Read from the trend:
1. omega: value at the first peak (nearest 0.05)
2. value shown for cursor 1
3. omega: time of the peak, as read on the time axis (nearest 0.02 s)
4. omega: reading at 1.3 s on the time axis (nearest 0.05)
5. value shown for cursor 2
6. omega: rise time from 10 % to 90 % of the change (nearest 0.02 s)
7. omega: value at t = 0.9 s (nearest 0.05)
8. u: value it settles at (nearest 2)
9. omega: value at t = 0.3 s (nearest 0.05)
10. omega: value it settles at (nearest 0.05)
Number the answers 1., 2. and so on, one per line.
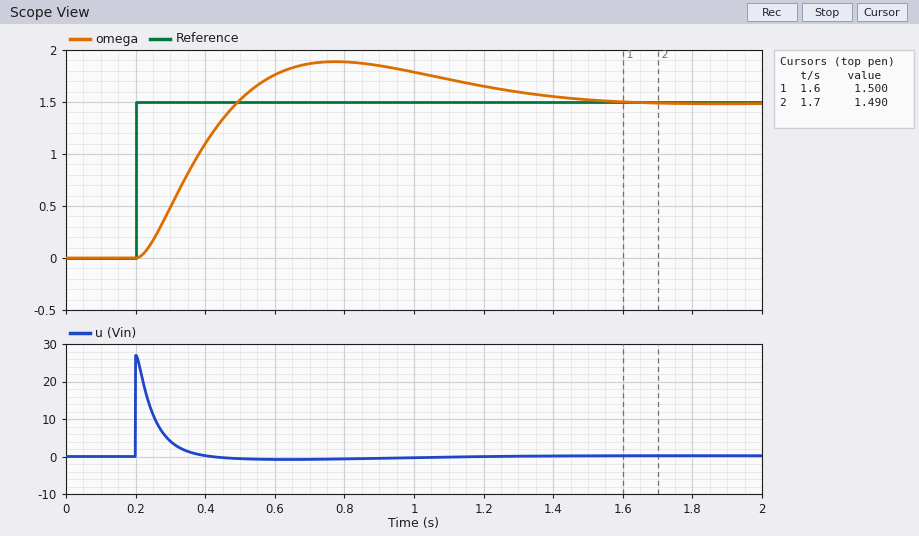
1. 1.90
2. 1.500
3. 0.78 s
4. 1.60
5. 1.490
6. 0.20 s
7. 1.85
8. 0
9. 0.50
10. 1.50
